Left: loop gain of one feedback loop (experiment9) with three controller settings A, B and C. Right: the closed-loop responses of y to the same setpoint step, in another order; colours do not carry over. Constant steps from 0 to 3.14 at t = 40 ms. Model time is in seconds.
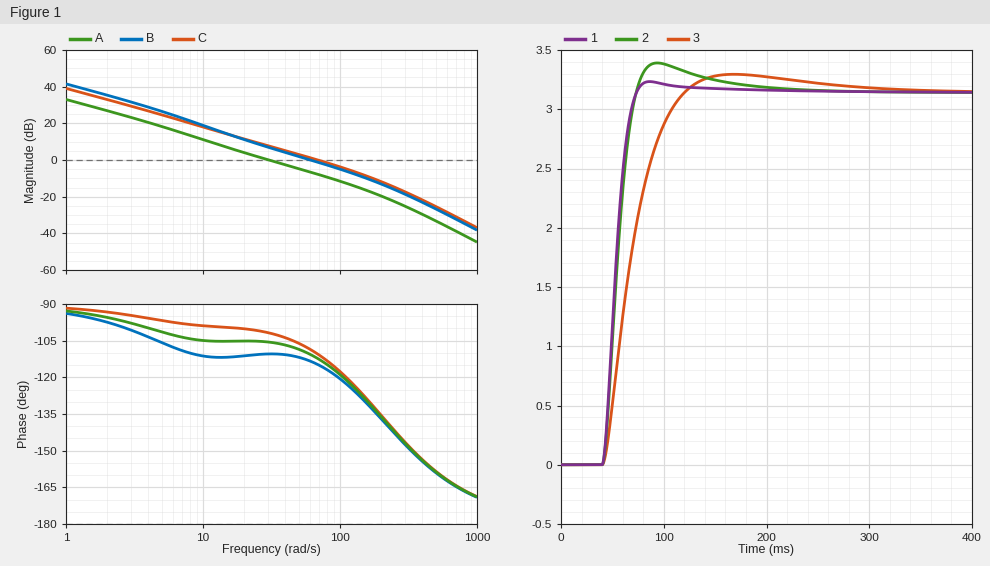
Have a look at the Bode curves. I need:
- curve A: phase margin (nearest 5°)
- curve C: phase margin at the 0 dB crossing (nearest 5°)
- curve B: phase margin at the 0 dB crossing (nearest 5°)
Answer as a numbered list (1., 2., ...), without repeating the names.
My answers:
1. 75°
2. 70°
3. 65°
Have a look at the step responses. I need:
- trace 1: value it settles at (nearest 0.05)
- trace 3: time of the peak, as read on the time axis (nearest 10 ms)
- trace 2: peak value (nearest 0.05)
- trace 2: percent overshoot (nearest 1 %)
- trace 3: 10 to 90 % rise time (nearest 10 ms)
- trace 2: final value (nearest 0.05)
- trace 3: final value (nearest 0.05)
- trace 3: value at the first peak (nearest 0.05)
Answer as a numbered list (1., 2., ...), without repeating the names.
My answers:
1. 3.15
2. 170 ms
3. 3.40
4. 8 %
5. 50 ms
6. 3.15
7. 3.15
8. 3.30
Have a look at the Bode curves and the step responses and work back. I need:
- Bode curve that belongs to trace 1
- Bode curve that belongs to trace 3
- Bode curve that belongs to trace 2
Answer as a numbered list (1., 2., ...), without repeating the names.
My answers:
1. C
2. A
3. B
